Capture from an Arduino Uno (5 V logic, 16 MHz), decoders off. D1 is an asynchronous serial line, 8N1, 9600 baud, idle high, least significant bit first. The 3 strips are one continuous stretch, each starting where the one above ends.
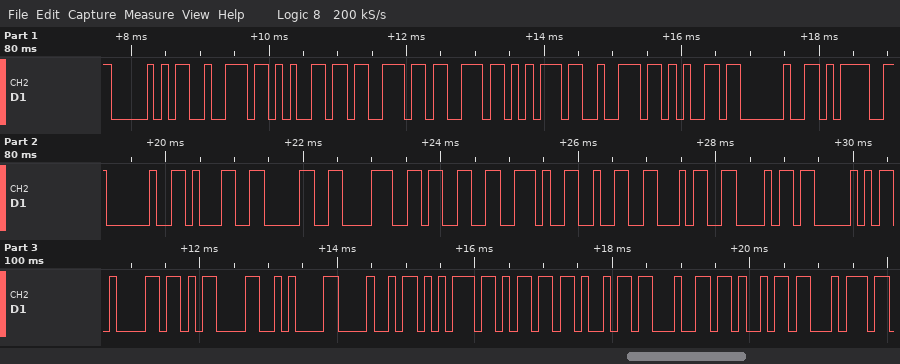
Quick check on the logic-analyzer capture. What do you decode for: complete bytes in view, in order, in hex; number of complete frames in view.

50 72 65 73 73 75 72 65 20 3D 20 31 30 38 33 2E 32 34 68 50 61 0D 0A 48 75 6D 69 64 69 74
30
